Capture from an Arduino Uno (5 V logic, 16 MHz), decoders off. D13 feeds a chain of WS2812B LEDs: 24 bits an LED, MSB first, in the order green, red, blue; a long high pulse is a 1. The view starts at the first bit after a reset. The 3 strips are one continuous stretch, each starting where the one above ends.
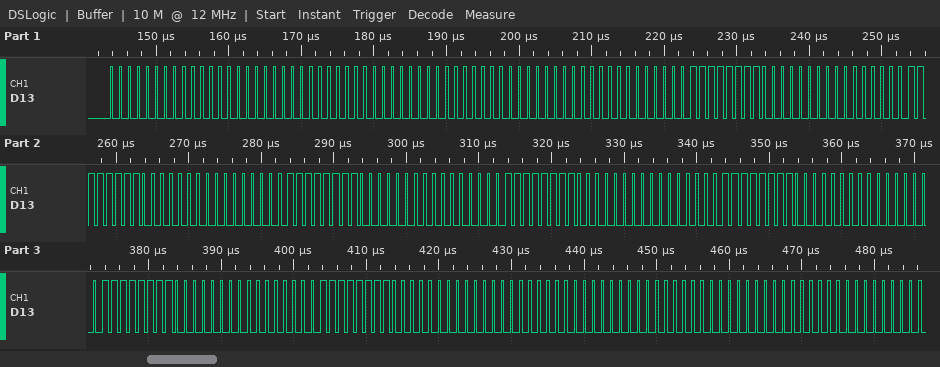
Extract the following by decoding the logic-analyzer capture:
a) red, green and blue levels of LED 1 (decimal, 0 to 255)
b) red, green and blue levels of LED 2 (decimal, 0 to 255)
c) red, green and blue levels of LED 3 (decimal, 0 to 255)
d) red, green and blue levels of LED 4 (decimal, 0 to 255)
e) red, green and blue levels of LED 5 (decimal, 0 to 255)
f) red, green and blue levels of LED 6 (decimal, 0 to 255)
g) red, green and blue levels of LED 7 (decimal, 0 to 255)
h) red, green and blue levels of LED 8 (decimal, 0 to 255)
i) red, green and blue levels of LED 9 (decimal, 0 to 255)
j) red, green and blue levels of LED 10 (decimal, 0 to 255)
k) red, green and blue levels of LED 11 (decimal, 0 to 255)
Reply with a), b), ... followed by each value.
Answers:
a) 0, 0, 0
b) 0, 0, 0
c) 0, 0, 255
d) 0, 0, 255
e) 0, 0, 255
f) 0, 0, 255
g) 0, 0, 255
h) 0, 0, 255
i) 0, 0, 255
j) 0, 0, 0
k) 0, 0, 0
